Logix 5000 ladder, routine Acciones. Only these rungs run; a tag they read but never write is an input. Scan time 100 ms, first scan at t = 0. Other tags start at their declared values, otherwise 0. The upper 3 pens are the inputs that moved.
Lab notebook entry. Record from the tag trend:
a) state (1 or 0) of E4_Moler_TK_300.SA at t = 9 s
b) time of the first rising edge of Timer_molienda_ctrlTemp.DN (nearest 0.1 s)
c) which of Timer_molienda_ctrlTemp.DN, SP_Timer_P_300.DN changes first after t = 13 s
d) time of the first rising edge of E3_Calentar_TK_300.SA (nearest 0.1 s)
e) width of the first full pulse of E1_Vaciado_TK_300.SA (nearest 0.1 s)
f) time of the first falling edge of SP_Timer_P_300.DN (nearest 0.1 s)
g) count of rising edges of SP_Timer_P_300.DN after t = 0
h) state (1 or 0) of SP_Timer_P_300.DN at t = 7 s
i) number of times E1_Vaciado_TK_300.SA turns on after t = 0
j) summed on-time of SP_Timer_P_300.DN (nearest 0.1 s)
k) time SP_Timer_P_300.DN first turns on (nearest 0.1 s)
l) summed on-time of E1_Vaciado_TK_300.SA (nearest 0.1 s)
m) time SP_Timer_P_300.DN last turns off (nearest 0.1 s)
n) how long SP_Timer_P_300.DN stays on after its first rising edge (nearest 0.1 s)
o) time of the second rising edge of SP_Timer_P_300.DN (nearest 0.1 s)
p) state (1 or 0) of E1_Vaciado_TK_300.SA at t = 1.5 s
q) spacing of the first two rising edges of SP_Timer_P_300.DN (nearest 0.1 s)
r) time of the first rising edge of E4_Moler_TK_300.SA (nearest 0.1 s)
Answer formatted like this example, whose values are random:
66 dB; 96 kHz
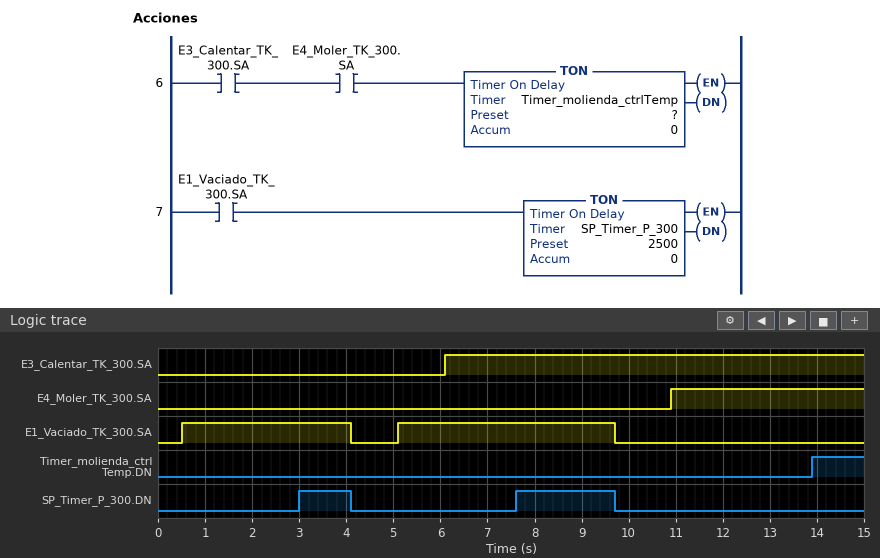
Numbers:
0; 13.9 s; Timer_molienda_ctrlTemp.DN; 6.1 s; 3.6 s; 4.1 s; 2; 0; 2; 3.2 s; 3.0 s; 8.2 s; 9.7 s; 1.1 s; 7.6 s; 1; 4.6 s; 10.9 s
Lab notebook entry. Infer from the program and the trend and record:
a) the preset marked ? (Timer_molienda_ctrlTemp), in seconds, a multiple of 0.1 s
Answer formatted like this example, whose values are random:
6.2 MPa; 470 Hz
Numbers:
3.0 s
